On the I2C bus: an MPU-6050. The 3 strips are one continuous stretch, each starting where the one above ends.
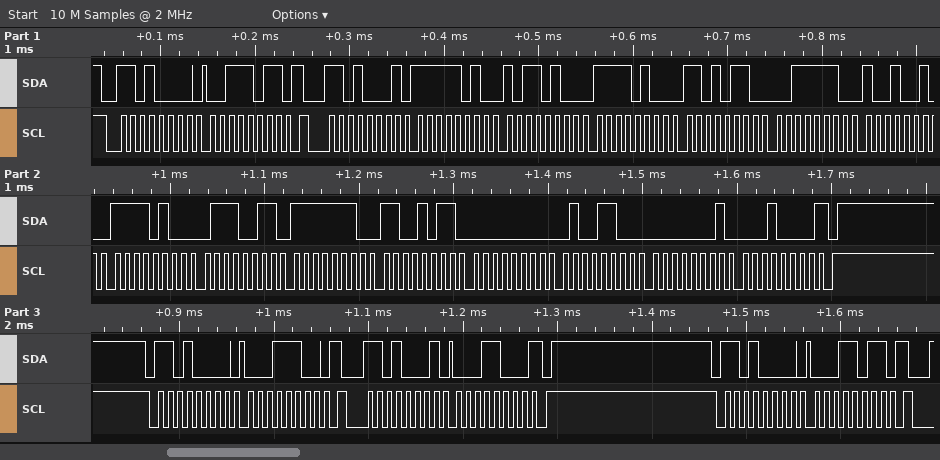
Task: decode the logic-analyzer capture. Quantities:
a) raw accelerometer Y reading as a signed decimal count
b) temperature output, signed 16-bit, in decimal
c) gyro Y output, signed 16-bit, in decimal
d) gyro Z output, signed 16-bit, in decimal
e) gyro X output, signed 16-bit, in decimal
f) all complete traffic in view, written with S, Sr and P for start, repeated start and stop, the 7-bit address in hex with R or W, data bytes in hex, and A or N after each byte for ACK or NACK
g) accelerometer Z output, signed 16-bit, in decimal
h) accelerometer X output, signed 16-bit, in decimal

-2858
-2957
76
272
-309
S 68W A 3B A Sr 68R A FA A B4 A F4 A D6 A 3E A 92 A F4 A 73 A FE A CB A 00 A 4C A 01 A 10 N P S 68W A 1C A Sr 68R A 18 N P S 68W A 1B A
16018
-1356
